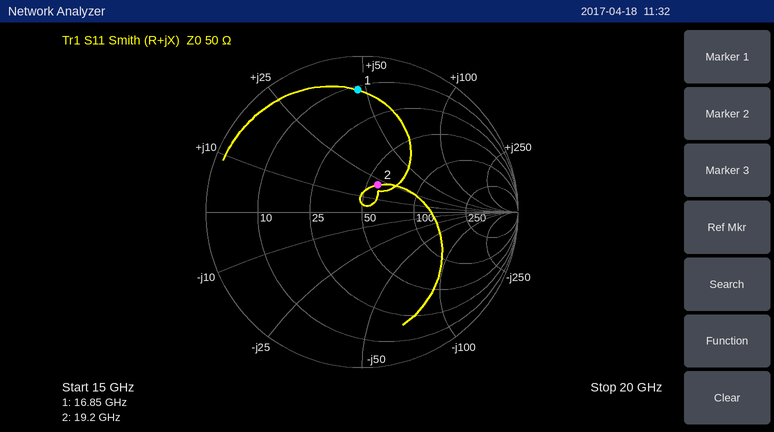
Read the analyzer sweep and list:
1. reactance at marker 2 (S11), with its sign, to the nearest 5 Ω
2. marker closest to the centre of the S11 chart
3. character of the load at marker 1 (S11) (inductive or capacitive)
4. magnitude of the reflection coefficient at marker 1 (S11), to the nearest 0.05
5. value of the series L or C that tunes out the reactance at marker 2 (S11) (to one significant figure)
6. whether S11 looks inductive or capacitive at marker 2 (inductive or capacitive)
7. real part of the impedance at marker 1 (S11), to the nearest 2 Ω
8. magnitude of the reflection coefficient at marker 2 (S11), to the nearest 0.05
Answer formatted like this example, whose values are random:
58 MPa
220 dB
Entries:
+20 Ω
marker 2
inductive
0.80
400 fF
inductive
12 Ω
0.20
